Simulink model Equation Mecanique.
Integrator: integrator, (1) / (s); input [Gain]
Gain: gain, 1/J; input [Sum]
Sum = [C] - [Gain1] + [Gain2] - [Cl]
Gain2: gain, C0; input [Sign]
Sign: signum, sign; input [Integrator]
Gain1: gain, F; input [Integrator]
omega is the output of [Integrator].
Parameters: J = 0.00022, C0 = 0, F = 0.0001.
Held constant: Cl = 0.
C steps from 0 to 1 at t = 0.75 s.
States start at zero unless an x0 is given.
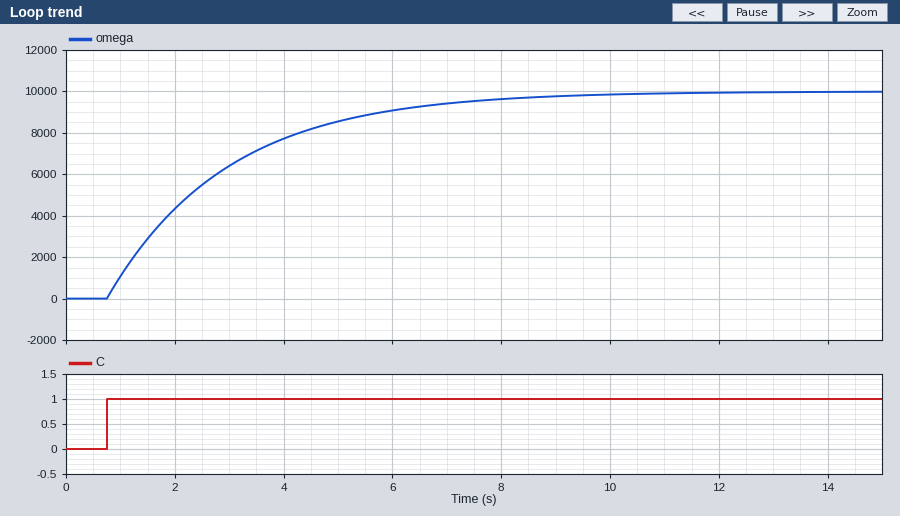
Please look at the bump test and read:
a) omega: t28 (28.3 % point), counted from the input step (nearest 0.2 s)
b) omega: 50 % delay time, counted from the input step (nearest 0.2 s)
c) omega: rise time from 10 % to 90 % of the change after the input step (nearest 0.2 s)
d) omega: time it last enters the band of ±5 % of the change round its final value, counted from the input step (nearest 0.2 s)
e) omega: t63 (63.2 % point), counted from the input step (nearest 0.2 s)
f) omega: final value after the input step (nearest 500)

0.8 s
1.6 s
4.8 s
6.6 s
2.2 s
10000
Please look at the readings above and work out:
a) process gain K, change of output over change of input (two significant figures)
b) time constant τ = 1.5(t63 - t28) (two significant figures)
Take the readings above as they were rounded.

10000
2.1 s
